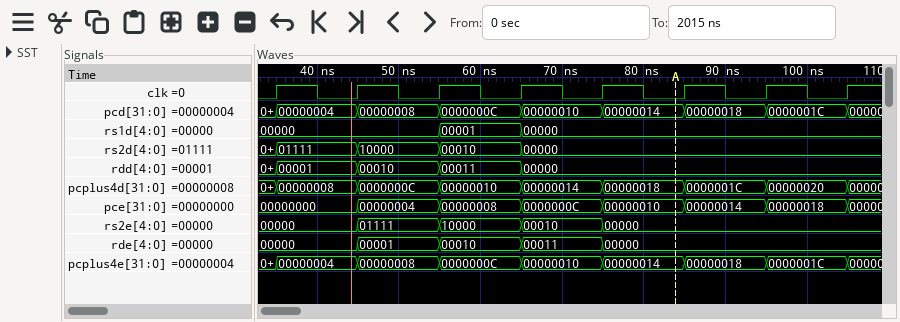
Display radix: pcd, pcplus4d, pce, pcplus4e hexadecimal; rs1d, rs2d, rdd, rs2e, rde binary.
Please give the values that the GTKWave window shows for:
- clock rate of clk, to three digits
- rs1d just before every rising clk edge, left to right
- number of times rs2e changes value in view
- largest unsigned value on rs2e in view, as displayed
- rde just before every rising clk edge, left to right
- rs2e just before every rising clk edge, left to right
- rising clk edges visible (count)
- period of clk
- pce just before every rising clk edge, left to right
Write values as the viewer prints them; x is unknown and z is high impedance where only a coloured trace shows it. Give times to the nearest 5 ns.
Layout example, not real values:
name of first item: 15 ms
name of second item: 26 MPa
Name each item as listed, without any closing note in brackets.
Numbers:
clock rate of clk, to three digits: 100 MHz
rs1d just before every rising clk edge, left to right: 00000, 00000, 00000, 00001, 00000, 00000, 00000, 00000
number of times rs2e changes value in view: 4
largest unsigned value on rs2e in view, as displayed: 10000
rde just before every rising clk edge, left to right: 00000, 00000, 00001, 00010, 00011, 00000, 00000, 00000
rs2e just before every rising clk edge, left to right: 00000, 00000, 01111, 10000, 00010, 00000, 00000, 00000
rising clk edges visible: 8
period of clk: 10 ns
pce just before every rising clk edge, left to right: 00000000, 00000000, 00000004, 00000008, 0000000C, 00000010, 00000014, 00000018
